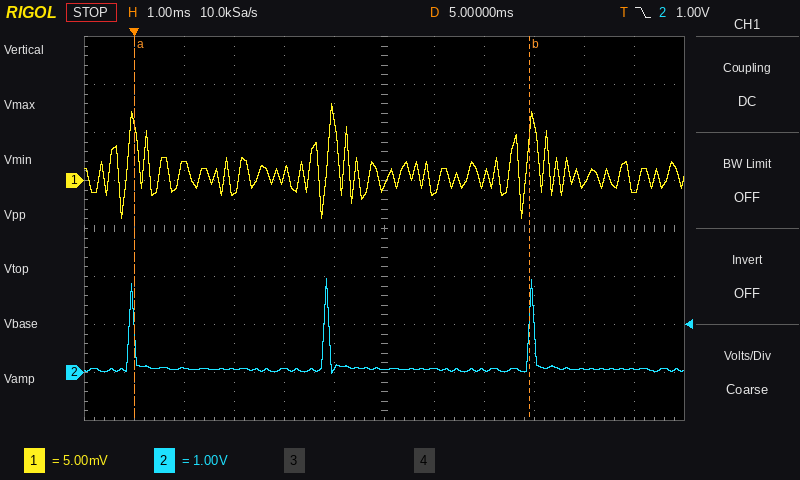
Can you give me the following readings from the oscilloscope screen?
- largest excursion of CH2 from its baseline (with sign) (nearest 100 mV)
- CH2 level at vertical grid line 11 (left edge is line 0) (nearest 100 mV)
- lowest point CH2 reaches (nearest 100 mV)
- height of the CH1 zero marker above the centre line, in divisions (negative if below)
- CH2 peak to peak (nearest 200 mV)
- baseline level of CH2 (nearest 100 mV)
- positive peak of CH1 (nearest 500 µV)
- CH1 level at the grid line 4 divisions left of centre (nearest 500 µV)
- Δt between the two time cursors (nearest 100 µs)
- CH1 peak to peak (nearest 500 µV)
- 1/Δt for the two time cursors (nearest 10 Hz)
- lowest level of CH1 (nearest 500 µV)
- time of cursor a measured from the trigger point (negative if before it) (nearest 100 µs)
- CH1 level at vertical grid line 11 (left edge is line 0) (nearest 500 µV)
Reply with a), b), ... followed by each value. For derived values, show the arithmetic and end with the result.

a) +1.9 V
b) 100 mV
c) 0.0 V
d) +1.0 div
e) 2.0 V
f) 100 mV
g) 8.0 mV
h) 2.0 mV
i) 7.9 ms
j) 8.0 mV − (-4.0 mV) = 12.0 mV
k) 1 / 7.9 ms ≈ 130 Hz
l) -4.0 mV
m) 0.0 ms
n) -1.0 mV
